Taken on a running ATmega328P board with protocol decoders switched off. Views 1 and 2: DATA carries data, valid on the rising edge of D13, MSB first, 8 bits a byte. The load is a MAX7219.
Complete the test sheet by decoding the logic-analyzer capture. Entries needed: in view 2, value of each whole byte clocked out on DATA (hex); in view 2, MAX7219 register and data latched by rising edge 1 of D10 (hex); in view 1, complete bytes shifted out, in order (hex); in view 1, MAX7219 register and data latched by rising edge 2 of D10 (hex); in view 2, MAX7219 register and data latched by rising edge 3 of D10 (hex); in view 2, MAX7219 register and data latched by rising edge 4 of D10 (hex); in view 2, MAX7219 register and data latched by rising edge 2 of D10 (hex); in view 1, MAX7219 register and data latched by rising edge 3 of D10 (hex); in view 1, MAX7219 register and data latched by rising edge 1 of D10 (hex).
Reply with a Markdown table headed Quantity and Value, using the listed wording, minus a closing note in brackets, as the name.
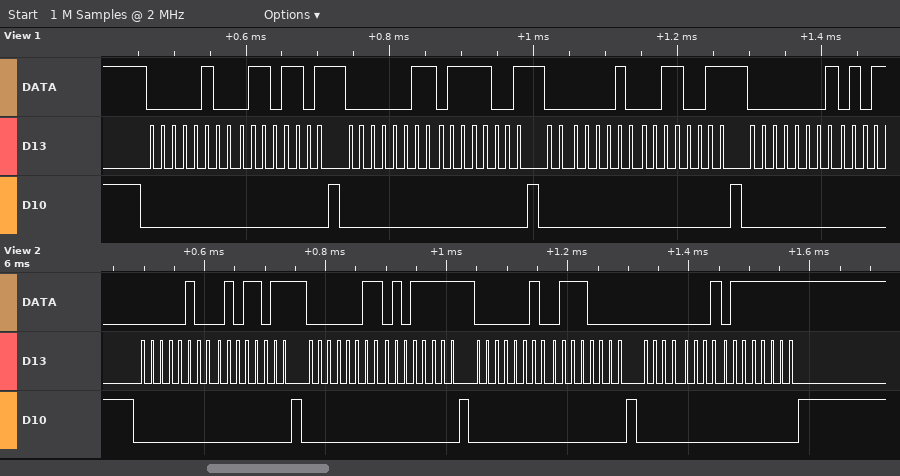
| Quantity | Value |
|---|---|
| in view 2, value of each whole byte clocked out on DATA | 04 5B 03 5F 02 70 01 7F |
| in view 2, MAX7219 register and data latched by rising edge 1 of D10 | register 0x4, data 0x5B |
| in view 1, complete bytes shifted out, in order | 04 6D 03 79 02 33 01 |
| in view 1, MAX7219 register and data latched by rising edge 2 of D10 | register 0x3, data 0x79 |
| in view 2, MAX7219 register and data latched by rising edge 3 of D10 | register 0x2, data 0x70 |
| in view 2, MAX7219 register and data latched by rising edge 4 of D10 | register 0x1, data 0x7F |
| in view 2, MAX7219 register and data latched by rising edge 2 of D10 | register 0x3, data 0x5F |
| in view 1, MAX7219 register and data latched by rising edge 3 of D10 | register 0x2, data 0x33 |
| in view 1, MAX7219 register and data latched by rising edge 1 of D10 | register 0x4, data 0x6D |
